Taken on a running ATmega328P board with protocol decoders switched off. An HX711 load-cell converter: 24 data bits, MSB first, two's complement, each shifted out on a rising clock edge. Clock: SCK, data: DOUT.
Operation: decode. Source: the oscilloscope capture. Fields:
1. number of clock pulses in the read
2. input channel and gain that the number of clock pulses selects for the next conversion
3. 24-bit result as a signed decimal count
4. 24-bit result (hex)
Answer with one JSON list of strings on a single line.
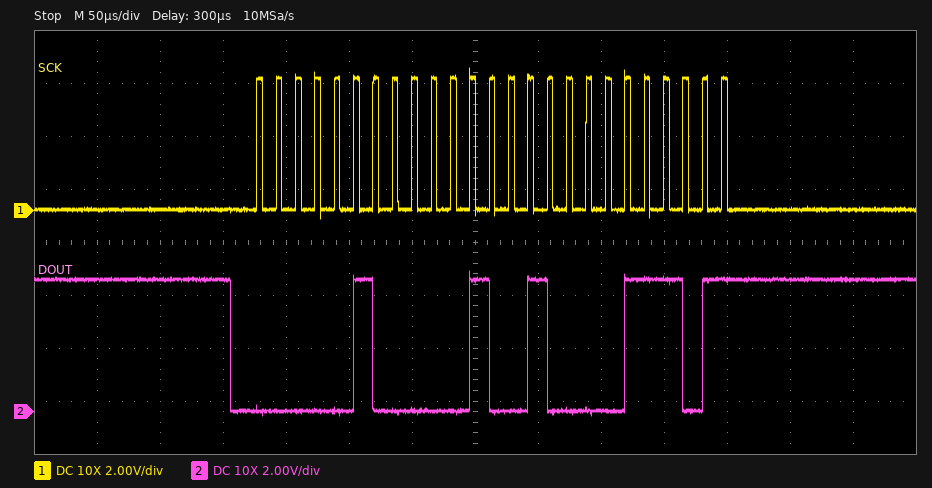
["25", "channel A, gain 128", "266781", "0x04121D"]
